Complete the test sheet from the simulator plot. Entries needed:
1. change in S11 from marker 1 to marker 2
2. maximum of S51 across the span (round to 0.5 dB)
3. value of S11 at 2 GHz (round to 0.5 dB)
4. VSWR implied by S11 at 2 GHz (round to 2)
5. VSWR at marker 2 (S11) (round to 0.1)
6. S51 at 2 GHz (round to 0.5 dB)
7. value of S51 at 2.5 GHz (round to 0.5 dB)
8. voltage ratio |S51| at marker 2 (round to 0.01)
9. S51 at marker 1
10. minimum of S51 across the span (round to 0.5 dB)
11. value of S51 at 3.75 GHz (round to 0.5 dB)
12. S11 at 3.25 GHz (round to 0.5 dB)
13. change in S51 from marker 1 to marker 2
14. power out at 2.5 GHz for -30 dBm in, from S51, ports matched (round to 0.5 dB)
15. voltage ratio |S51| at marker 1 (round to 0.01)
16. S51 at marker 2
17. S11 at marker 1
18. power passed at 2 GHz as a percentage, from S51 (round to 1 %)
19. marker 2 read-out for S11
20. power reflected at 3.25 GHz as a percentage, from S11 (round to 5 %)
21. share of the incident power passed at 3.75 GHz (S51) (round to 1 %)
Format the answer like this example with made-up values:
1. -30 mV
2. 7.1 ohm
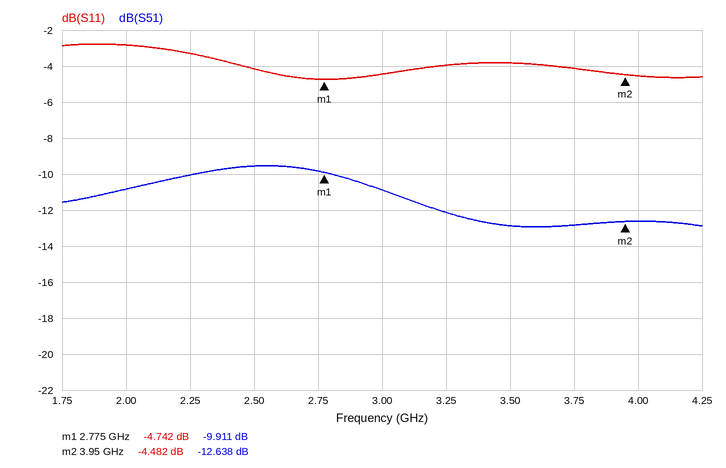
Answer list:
1. 0.260 dB
2. -9.5 dB
3. -3.0 dB
4. 6
5. 4.0
6. -11.0 dB
7. -9.5 dB
8. 0.23
9. -9.911 dB
10. -13.0 dB
11. -13.0 dB
12. -4.0 dB
13. -2.727 dB
14. -39.5 dBm
15. 0.32
16. -12.638 dB
17. -4.742 dB
18. 8 %
19. -4.482 dB
20. 40 %
21. 5 %
